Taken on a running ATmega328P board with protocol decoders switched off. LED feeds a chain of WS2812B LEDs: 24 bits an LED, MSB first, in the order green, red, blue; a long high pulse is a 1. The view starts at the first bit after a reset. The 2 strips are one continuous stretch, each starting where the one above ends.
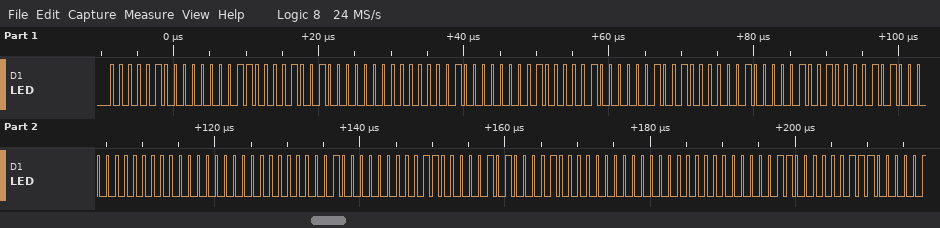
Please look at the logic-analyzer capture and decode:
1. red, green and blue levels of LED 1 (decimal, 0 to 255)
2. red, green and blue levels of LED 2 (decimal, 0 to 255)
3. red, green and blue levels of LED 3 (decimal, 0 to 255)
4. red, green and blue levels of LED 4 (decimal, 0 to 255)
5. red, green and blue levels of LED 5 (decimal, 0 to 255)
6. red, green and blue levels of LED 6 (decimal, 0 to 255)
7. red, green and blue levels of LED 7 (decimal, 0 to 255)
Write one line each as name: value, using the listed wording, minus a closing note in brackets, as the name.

red, green and blue levels of LED 1: 3, 4, 9
red, green and blue levels of LED 2: 2, 0, 1
red, green and blue levels of LED 3: 9, 4, 2
red, green and blue levels of LED 4: 10, 9, 0
red, green and blue levels of LED 5: 0, 0, 8
red, green and blue levels of LED 6: 5, 3, 8
red, green and blue levels of LED 7: 0, 0, 6
